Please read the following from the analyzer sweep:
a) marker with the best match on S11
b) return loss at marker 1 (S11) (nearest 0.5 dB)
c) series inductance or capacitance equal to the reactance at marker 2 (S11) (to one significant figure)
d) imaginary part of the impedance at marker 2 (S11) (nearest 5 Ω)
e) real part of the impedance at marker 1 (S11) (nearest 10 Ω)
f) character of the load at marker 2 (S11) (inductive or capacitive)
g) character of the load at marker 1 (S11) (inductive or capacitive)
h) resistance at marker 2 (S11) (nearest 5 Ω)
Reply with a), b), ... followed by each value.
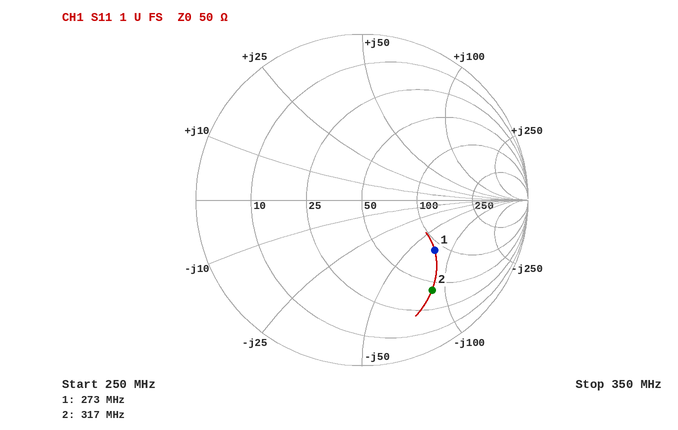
a) marker 1
b) 5.5 dB
c) 6 pF
d) -85 Ω
e) 90 Ω
f) capacitive
g) capacitive
h) 40 Ω
